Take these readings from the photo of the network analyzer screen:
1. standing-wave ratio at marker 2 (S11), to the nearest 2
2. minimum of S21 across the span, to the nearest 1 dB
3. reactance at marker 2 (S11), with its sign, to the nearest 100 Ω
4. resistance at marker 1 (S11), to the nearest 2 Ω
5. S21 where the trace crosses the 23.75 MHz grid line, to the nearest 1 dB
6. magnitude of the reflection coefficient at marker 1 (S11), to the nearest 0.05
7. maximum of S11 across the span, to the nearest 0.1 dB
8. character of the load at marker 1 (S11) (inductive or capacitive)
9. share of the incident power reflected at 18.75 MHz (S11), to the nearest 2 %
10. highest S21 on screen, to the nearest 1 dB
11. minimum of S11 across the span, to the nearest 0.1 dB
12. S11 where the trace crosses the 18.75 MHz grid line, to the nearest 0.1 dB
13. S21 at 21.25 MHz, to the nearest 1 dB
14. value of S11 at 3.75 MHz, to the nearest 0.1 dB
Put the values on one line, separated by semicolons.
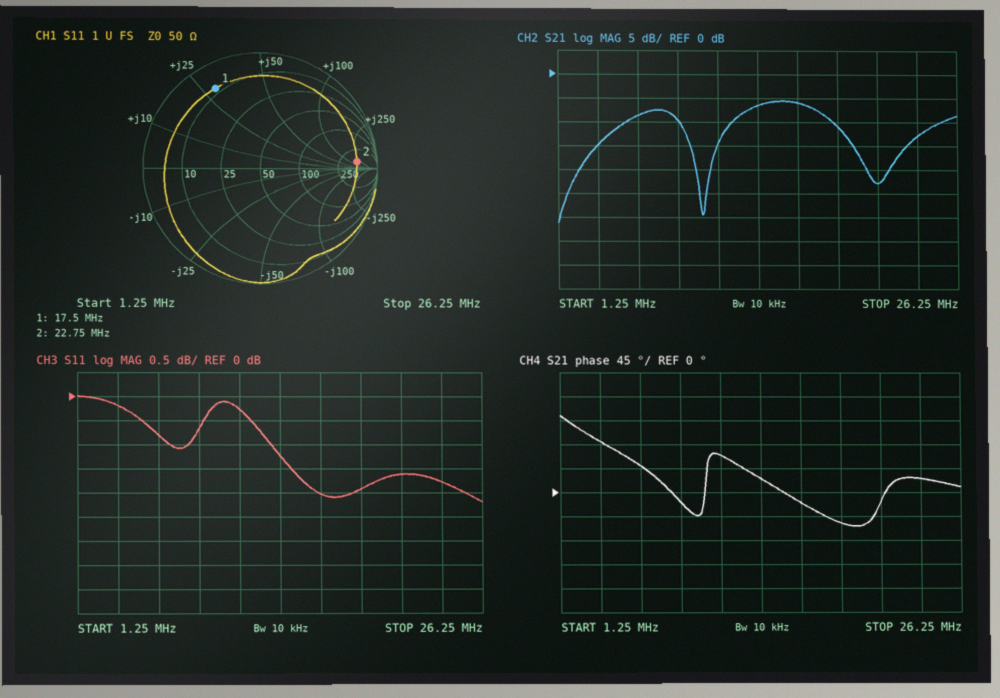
10; -31 dB; +200 Ω; 8 Ω; -13 dB; 0.80; 0.0 dB; inductive; 64 %; -6 dB; -2.2 dB; -1.9 dB; -23 dB; -0.2 dB
